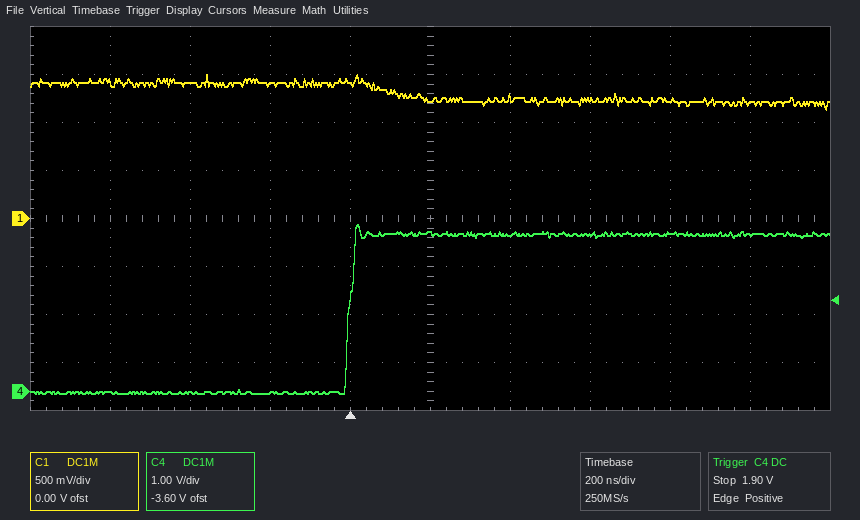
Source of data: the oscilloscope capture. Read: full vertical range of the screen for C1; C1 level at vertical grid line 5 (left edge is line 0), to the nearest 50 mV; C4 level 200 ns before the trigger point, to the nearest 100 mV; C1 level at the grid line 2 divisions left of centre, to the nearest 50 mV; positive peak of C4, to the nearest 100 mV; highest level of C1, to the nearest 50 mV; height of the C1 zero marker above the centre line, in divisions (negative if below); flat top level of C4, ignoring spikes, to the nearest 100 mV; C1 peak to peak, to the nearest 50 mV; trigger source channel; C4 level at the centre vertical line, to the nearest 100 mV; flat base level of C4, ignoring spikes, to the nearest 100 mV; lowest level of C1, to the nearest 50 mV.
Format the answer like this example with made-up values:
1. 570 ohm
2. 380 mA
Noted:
1. 4 V
2. 1.25 V
3. 0.0 V
4. 1.40 V
5. 3.5 V
6. 1.50 V
7. 0.0 div
8. 3.3 V
9. 350 mV
10. C4
11. 3.3 V
12. 0.0 V
13. 1.15 V
